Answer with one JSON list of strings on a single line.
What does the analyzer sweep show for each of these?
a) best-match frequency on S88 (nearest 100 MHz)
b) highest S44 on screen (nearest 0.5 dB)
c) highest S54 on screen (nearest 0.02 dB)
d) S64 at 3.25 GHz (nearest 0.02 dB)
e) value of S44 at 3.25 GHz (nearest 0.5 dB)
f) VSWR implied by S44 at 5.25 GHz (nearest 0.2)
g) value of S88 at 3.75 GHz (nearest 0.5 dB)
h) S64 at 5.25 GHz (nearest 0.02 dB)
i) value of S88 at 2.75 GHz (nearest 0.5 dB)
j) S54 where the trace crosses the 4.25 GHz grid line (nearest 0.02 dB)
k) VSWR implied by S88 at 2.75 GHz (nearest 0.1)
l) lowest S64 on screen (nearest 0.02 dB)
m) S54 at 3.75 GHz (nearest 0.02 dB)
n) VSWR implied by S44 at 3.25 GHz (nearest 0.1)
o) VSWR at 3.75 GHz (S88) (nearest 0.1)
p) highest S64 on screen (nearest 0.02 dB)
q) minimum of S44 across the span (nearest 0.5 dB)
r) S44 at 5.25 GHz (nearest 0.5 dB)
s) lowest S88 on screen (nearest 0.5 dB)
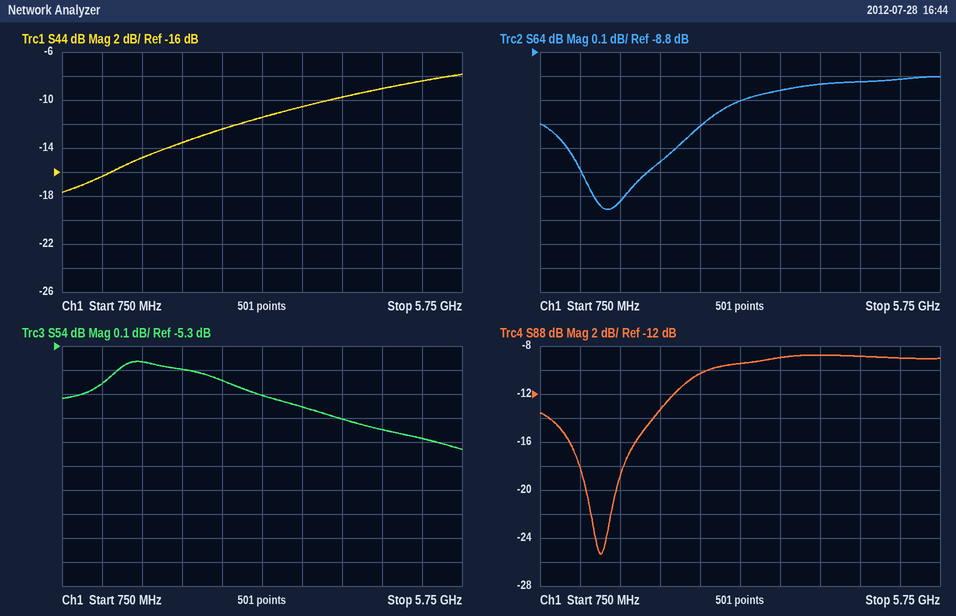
["1.5 GHz", "-8.0 dB", "-5.36 dB", "-9.00 dB", "-11.5 dB", "2.2", "-9.0 dB", "-8.92 dB", "-10.5 dB", "-5.60 dB", "1.9", "-9.46 dB", "-5.56 dB", "1.7", "2.1", "-8.90 dB", "-17.5 dB", "-8.5 dB", "-25.5 dB"]
